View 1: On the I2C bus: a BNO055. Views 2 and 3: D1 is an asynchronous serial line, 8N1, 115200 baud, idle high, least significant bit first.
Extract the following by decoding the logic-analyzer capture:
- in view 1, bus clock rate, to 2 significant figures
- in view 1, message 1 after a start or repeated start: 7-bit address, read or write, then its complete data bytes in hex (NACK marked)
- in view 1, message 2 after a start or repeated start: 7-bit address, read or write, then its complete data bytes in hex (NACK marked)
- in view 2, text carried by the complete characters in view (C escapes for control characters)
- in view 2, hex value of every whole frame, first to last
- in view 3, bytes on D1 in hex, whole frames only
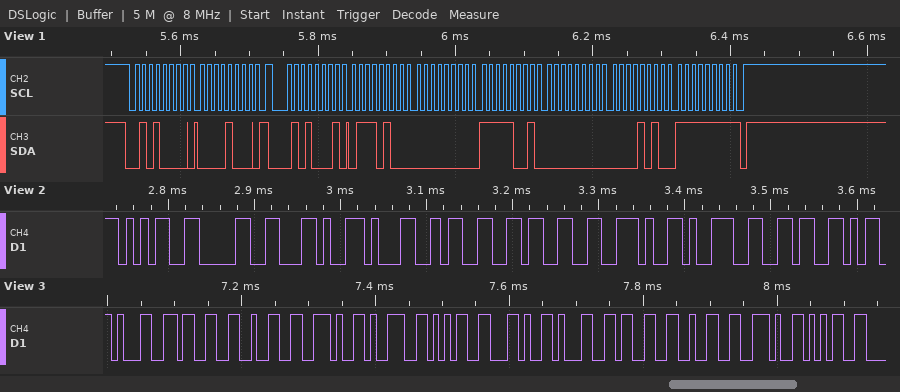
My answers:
100 kHz
0x28 write: 08
0x28 read: 74 00 F9 00 0A FF NACK
"50,133.96"
35 30 2C 31 33 33 2E 39 36
0x31 0x33 0x32 0x2E 0x39 0x35 0x2C 0x31 0x33 0x32 0x2E 0x35
